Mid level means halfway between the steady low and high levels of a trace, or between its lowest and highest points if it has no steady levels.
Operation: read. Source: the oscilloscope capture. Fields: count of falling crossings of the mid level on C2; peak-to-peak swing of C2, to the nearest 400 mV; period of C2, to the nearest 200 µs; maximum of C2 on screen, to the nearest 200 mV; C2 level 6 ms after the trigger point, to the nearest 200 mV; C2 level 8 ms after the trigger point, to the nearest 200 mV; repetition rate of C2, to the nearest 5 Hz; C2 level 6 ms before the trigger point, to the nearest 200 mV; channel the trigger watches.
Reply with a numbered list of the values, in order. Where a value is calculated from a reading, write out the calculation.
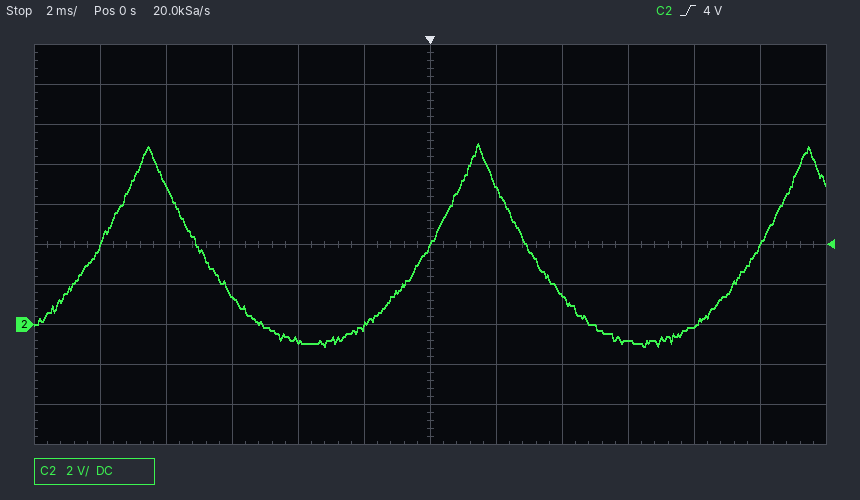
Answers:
1. 2
2. 10.0 V
3. 10.0 ms
4. 9.0 V
5. -800 mV
6. 0.0 V
7. 1 / 10.0 ms ≈ 100 Hz
8. 1.4 V
9. C2
